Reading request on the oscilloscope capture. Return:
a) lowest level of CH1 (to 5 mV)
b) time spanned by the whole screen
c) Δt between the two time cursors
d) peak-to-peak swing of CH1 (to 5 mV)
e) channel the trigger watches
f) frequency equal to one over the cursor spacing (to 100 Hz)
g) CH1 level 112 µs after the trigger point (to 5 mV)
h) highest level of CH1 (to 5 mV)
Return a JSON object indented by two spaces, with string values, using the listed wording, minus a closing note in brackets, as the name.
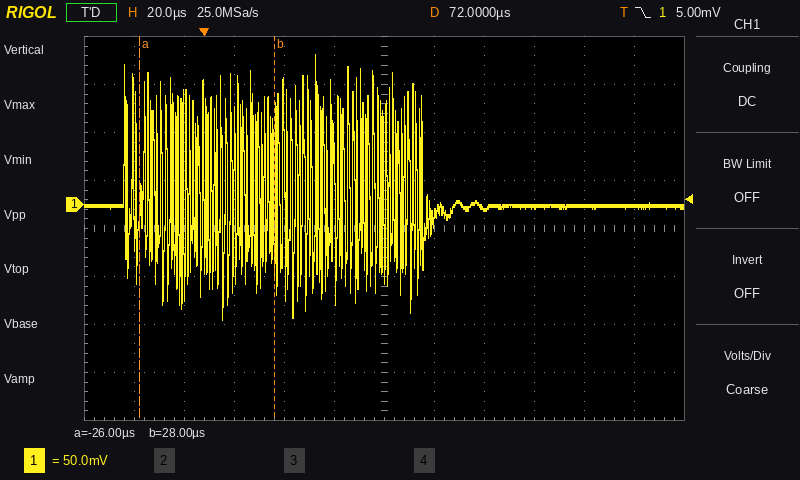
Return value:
{
  "lowest level of CH1": "-120 mV",
  "time spanned by the whole screen": "240 µs",
  "Δt between the two time cursors": "54 µs",
  "peak-to-peak swing of CH1": "275 mV",
  "channel the trigger watches": "CH1",
  "frequency equal to one over the cursor spacing": "18.5 kHz",
  "CH1 level 112 µs after the trigger point": "-5 mV",
  "highest level of CH1": "155 mV"
}
